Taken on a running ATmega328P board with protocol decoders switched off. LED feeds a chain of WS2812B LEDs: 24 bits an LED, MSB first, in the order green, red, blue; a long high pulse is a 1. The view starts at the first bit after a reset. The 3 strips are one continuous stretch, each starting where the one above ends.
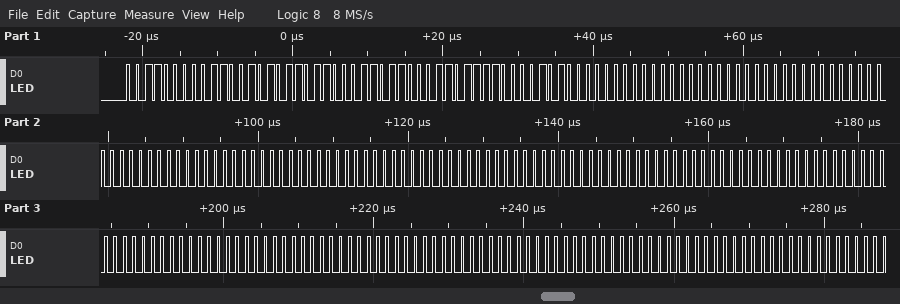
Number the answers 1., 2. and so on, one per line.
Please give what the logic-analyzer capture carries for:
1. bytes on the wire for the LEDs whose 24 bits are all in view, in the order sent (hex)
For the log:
1. 30 65 6C 6C 6F 0A 00 00 00 00 00 00 00 00 00 00 00 00 00 00 00 00 00 00 00 00 00 00 00 00
